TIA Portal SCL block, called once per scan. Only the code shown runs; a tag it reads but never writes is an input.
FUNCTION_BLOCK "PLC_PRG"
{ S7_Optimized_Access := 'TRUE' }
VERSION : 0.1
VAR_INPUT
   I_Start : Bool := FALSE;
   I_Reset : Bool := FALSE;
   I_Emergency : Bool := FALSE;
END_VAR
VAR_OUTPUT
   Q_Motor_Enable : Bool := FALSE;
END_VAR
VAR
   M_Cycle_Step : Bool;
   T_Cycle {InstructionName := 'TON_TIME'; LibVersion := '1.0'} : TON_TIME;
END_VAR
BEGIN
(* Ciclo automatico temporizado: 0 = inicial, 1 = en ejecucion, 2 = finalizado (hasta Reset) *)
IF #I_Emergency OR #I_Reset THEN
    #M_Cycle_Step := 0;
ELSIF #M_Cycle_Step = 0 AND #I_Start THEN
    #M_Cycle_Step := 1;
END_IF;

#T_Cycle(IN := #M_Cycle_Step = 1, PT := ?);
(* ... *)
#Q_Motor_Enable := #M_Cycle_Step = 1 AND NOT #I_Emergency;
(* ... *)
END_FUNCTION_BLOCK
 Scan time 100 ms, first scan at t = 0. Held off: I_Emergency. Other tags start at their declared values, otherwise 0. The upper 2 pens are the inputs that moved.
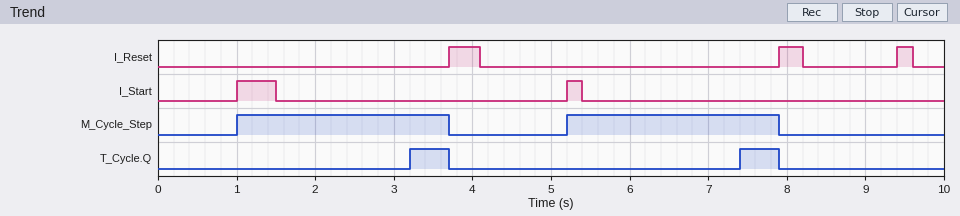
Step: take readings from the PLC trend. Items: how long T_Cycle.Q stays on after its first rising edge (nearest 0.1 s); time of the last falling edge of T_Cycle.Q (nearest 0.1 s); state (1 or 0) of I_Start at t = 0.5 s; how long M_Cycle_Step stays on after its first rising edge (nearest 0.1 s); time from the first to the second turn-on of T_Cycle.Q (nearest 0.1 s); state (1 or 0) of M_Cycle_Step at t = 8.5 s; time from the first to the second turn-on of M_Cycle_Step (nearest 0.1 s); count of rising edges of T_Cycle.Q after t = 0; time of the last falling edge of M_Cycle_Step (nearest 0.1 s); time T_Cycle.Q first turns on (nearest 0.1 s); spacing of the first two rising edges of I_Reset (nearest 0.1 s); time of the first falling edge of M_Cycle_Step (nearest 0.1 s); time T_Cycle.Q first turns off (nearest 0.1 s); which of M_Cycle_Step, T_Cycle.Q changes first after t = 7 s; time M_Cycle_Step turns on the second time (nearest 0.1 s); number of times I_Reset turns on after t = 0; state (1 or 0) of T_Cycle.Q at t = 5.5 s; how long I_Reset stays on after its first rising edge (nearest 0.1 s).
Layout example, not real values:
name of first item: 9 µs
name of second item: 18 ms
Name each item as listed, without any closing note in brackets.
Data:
how long T_Cycle.Q stays on after its first rising edge: 0.5 s
time of the last falling edge of T_Cycle.Q: 7.9 s
state (1 or 0) of I_Start at t = 0.5 s: 0
how long M_Cycle_Step stays on after its first rising edge: 2.7 s
time from the first to the second turn-on of T_Cycle.Q: 4.2 s
state (1 or 0) of M_Cycle_Step at t = 8.5 s: 0
time from the first to the second turn-on of M_Cycle_Step: 4.2 s
count of rising edges of T_Cycle.Q after t = 0: 2
time of the last falling edge of M_Cycle_Step: 7.9 s
time T_Cycle.Q first turns on: 3.2 s
spacing of the first two rising edges of I_Reset: 4.2 s
time of the first falling edge of M_Cycle_Step: 3.7 s
time T_Cycle.Q first turns off: 3.7 s
which of M_Cycle_Step, T_Cycle.Q changes first after t = 7 s: T_Cycle.Q
time M_Cycle_Step turns on the second time: 5.2 s
number of times I_Reset turns on after t = 0: 3
state (1 or 0) of T_Cycle.Q at t = 5.5 s: 0
how long I_Reset stays on after its first rising edge: 0.4 s
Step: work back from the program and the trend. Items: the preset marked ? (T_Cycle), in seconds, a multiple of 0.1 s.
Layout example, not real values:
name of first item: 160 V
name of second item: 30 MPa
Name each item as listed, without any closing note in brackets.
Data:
the preset marked ? (T_Cycle), in seconds, a multiple of 0.1 s: 2.2 s
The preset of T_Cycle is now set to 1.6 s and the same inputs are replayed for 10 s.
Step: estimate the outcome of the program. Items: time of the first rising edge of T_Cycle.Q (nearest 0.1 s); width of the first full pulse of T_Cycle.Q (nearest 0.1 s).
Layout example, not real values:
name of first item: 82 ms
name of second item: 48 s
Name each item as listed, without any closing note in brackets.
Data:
time of the first rising edge of T_Cycle.Q: 2.6 s
width of the first full pulse of T_Cycle.Q: 1.1 s
